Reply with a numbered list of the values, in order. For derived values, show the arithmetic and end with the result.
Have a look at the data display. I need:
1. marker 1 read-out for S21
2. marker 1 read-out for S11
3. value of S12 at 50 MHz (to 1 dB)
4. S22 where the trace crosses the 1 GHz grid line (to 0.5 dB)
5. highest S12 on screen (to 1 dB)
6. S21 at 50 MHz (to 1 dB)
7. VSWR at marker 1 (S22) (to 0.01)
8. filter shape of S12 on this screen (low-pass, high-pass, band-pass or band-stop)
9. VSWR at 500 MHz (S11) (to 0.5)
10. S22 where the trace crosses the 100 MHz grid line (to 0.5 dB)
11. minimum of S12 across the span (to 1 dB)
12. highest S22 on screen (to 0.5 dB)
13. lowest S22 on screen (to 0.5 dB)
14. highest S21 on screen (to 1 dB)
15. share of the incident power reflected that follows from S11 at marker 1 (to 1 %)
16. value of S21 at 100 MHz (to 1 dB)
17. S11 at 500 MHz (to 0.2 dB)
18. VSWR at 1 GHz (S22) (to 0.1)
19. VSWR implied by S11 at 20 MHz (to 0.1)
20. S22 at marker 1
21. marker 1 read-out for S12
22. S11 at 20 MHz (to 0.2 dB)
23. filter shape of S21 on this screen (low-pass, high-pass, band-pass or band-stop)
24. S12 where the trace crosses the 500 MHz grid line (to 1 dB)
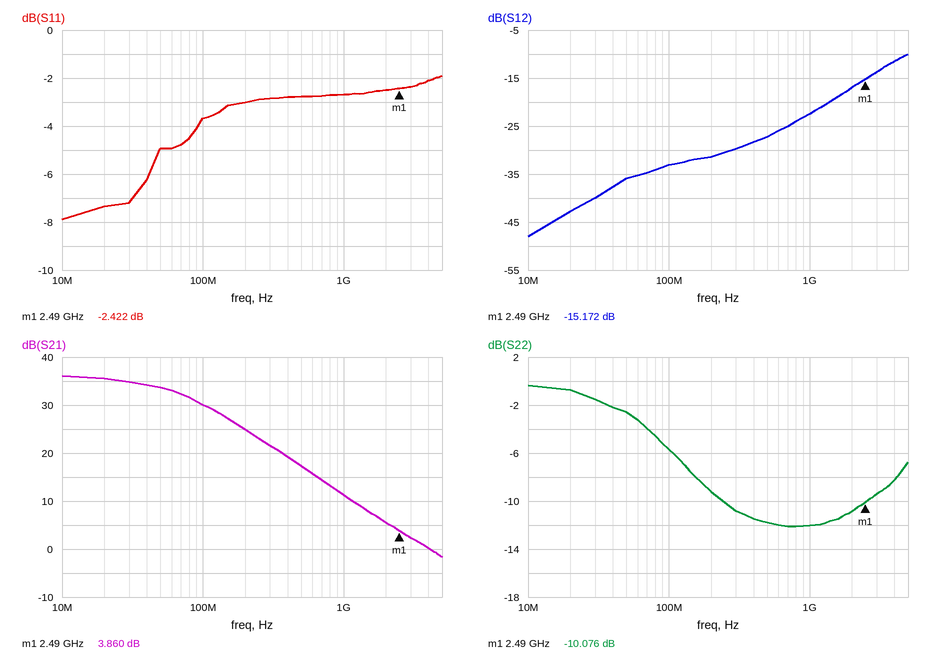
1. 3.860 dB
2. -2.422 dB
3. -36 dB
4. -12.0 dB
5. -10 dB
6. 34 dB
7. (1 + 0.3135)/(1 − 0.3135) ≈ 1.91
8. high-pass
9. |Γ| = 10^(-2.8/20) = 0.7244; VSWR = (1 + 0.7244)/(1 − 0.7244) ≈ 6.26, so 6.5 to the nearest 0.5
10. -5.5 dB
11. -48 dB
12. -0.5 dB
13. -12.0 dB
14. 36 dB
15. 10^(-2.422/10) ≈ 57 %
16. 30 dB
17. -2.8 dB
18. |Γ| = 10^(-12/20) = 0.2512; VSWR = (1 + 0.2512)/(1 − 0.2512) ≈ 1.7
19. |Γ| = 10^(-7.4/20) = 0.4266; VSWR = (1 + 0.4266)/(1 − 0.4266) ≈ 2.5
20. -10.076 dB
21. -15.172 dB
22. -7.4 dB
23. low-pass
24. -27 dB
